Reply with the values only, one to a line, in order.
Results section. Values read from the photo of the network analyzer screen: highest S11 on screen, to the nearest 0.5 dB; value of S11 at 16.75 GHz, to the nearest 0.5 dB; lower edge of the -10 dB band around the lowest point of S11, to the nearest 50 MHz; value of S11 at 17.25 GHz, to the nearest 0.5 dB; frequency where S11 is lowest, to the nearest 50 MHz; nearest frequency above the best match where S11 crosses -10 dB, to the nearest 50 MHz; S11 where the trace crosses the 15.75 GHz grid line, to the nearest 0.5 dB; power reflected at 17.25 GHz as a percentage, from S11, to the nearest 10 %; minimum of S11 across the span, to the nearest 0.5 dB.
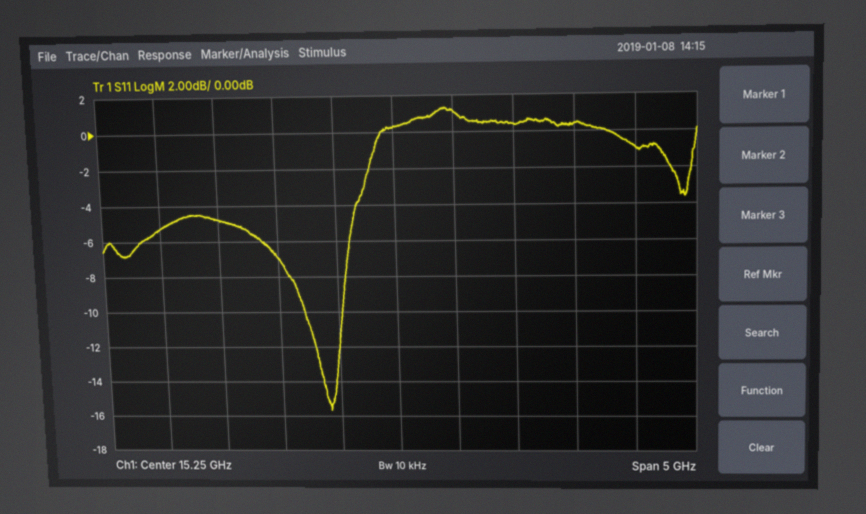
1.5 dB
0.5 dB
14.45 GHz
-1.0 dB
14.65 GHz
14.80 GHz
1.0 dB
80 %
-15.5 dB
